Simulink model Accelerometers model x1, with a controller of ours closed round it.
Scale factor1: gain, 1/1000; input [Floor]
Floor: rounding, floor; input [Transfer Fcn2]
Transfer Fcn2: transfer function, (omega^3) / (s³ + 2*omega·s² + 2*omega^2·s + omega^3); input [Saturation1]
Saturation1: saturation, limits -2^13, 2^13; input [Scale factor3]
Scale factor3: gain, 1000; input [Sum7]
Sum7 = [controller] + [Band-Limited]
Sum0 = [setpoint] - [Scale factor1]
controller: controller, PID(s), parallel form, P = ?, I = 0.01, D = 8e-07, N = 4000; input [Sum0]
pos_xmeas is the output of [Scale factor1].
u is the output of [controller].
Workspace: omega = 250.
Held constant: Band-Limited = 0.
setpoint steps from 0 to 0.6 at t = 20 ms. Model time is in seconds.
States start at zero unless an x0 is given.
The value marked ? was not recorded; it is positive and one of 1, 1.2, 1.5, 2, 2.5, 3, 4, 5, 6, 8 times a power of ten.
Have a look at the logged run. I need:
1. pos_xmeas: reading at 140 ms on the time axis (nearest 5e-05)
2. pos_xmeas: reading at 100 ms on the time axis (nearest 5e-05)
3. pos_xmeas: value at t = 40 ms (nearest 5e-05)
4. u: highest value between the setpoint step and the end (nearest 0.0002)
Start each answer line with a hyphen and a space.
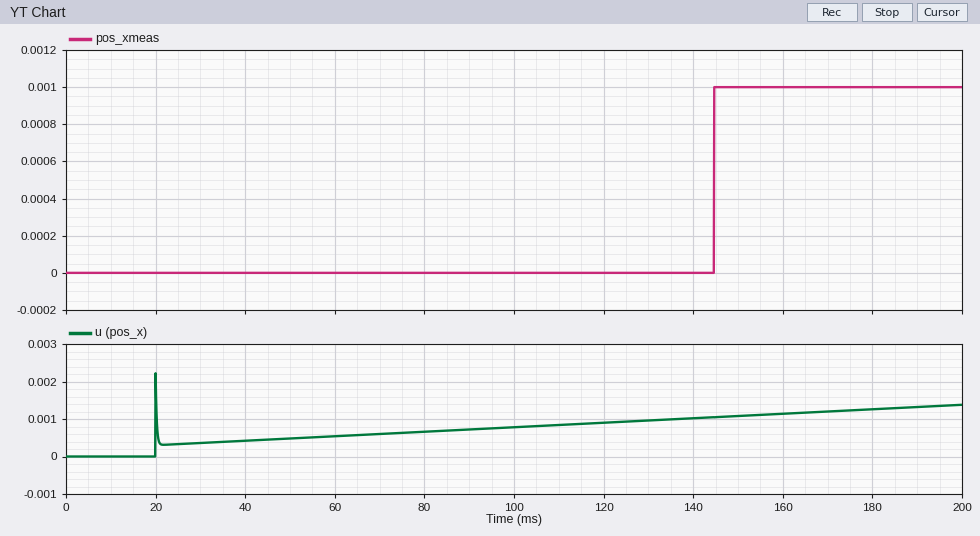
- 0.00000
- 0.00000
- 0.00000
- 0.0022
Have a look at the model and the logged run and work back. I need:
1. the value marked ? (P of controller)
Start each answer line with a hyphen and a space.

- 0.0005
